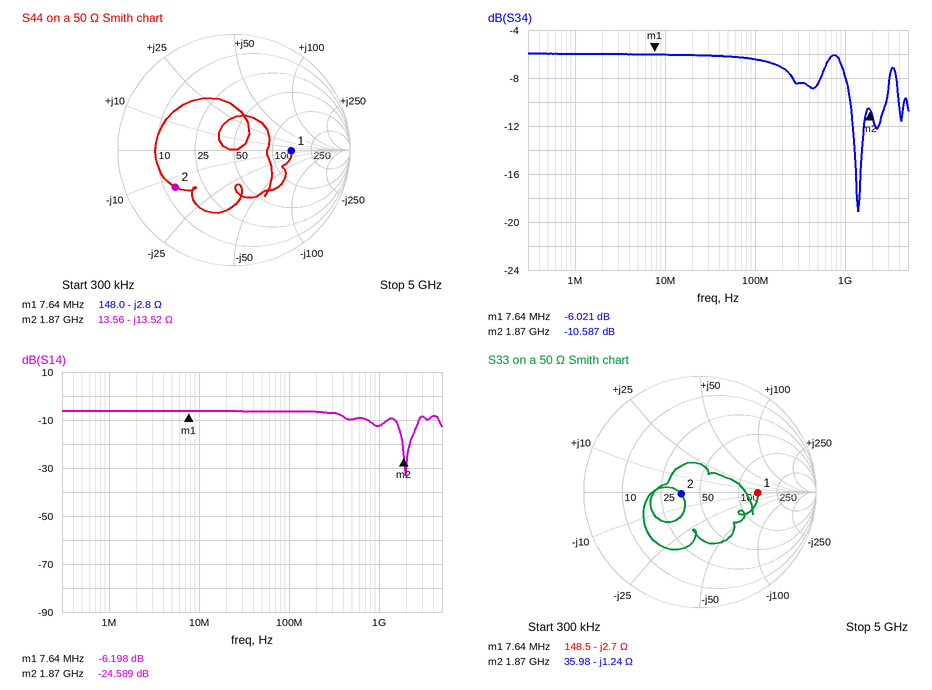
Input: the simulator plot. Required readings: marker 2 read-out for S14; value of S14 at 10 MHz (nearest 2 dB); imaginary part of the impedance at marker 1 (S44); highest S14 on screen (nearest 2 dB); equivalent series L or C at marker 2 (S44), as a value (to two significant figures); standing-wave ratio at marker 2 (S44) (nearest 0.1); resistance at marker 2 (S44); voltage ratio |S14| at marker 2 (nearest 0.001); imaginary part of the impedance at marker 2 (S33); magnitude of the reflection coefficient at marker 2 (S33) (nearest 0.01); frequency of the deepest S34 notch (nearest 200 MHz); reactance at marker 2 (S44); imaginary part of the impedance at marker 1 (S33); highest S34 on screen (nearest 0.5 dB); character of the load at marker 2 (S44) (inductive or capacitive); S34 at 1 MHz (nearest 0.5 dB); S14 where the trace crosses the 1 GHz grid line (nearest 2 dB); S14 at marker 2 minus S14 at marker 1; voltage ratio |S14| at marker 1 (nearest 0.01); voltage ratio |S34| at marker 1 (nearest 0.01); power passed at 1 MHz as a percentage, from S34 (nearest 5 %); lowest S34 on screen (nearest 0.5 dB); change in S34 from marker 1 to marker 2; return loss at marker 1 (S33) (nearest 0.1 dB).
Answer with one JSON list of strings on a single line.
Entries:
["-24.589 dB", "-6 dB", "-2.8 Ω", "-6 dB", "6.3 pF", "4.0", "13.56 Ω", "0.059", "-1.24 Ω", "0.16", "1.4 GHz", "-13.52 Ω", "-2.7 Ω", "-6.0 dB", "capacitive", "-6.0 dB", "-12 dB", "-18.391 dB", "0.49", "0.50", "25 %", "-19.0 dB", "-4.566 dB", "6.1 dB"]
